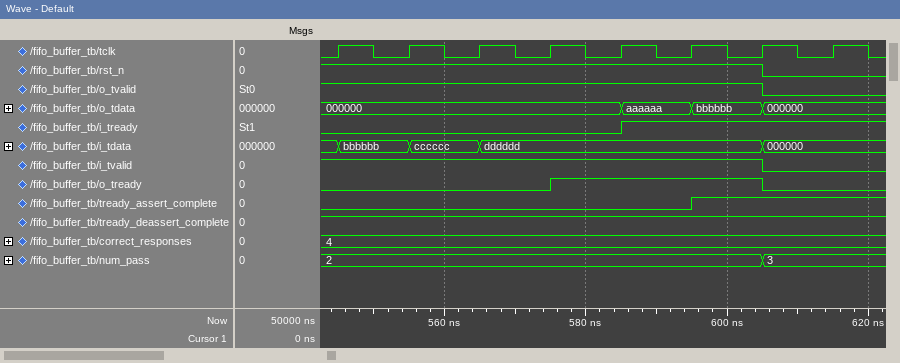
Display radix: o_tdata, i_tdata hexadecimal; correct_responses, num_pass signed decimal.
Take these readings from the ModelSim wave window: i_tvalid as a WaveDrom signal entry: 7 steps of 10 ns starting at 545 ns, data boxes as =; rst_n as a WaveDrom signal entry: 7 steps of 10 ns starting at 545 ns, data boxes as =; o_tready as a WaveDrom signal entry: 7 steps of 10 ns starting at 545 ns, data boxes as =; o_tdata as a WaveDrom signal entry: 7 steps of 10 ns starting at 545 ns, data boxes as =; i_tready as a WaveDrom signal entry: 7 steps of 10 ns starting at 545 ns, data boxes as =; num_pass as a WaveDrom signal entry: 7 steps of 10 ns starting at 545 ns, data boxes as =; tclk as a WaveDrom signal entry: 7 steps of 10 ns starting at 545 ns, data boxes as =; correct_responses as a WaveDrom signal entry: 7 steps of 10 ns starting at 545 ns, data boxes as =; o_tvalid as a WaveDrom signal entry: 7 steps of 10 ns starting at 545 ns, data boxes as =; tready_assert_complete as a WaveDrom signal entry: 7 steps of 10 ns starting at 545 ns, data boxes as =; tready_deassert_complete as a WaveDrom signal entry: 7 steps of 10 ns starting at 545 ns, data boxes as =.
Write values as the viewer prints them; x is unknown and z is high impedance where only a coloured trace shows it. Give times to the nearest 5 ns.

{name: 'i_tvalid', wave: '1.....0'}
{name: 'rst_n', wave: '1.....0'}
{name: 'o_tready', wave: '0..1..0'}
{name: 'o_tdata', wave: '=...===', data: '000000 aaaaaa bbbbbb 000000'}
{name: 'i_tready', wave: '0...1..'}
{name: 'num_pass', wave: '=.....=', data: '2 3'}
{name: 'tclk', wave: 'p......'}
{name: 'correct_responses', wave: '=......', data: '4'}
{name: 'o_tvalid', wave: '1.....0'}
{name: 'tready_assert_complete', wave: '0....1.'}
{name: 'tready_deassert_complete', wave: '1......'}
